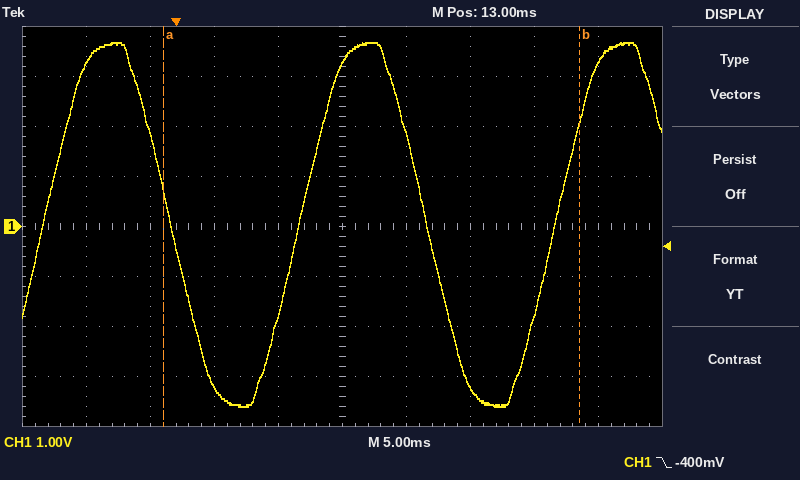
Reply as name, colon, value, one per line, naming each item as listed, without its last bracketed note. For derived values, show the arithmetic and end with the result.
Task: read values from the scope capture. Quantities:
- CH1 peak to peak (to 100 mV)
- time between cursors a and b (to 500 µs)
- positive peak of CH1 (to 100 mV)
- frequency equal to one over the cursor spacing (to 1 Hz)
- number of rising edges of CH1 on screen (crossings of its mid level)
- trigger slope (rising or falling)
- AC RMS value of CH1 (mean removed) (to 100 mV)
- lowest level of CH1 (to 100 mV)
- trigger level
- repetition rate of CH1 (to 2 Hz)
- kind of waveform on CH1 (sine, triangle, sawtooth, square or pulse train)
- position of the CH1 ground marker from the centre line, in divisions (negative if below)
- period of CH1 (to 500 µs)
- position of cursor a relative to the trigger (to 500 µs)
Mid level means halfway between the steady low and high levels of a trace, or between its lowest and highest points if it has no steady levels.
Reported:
CH1 peak to peak: 3.7 V − (-3.6 V) = 7.3 V
time between cursors a and b: 32.5 ms
positive peak of CH1: 3.7 V
frequency equal to one over the cursor spacing: 1 / 32.5 ms ≈ 31 Hz
number of rising edges of CH1 on screen: 3
trigger slope: falling
AC RMS value of CH1 (mean removed): 7.3 V / (2√2) ≈ 2.6 V
lowest level of CH1: -3.6 V
trigger level: -400 mV
repetition rate of CH1: 1 / 20.0 ms ≈ 50 Hz
kind of waveform on CH1: sine
position of the CH1 ground marker from the centre line, in divisions: 0.0 div
period of CH1: 20.0 ms
position of cursor a relative to the trigger: -1.0 ms
